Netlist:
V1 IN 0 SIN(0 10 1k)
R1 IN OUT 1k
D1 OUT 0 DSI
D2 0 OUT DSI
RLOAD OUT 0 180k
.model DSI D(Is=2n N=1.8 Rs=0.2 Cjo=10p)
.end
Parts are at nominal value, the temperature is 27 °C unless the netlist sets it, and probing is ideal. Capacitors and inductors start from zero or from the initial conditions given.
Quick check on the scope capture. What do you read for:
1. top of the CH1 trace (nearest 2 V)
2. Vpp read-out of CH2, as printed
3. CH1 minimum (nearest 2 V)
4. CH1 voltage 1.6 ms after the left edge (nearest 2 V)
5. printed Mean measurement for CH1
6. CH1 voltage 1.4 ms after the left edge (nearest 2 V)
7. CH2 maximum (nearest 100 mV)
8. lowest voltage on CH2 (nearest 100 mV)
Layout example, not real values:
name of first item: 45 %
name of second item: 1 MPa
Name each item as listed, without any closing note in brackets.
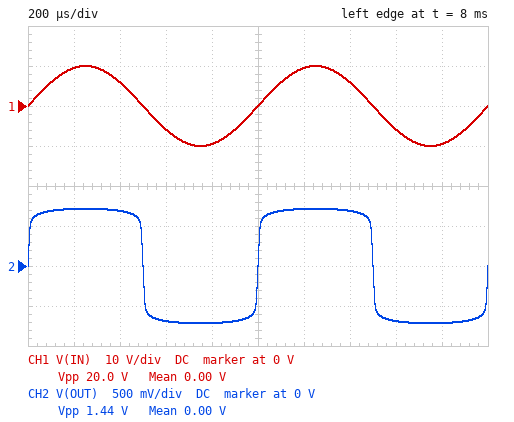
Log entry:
top of the CH1 trace: 10 V
Vpp read-out of CH2, as printed: 1.44 V
CH1 minimum: -10 V
CH1 voltage 1.6 ms after the left edge: -6 V
printed Mean measurement for CH1: 0.00 V
CH1 voltage 1.4 ms after the left edge: 6 V
CH2 maximum: 700 mV
lowest voltage on CH2: -700 mV
